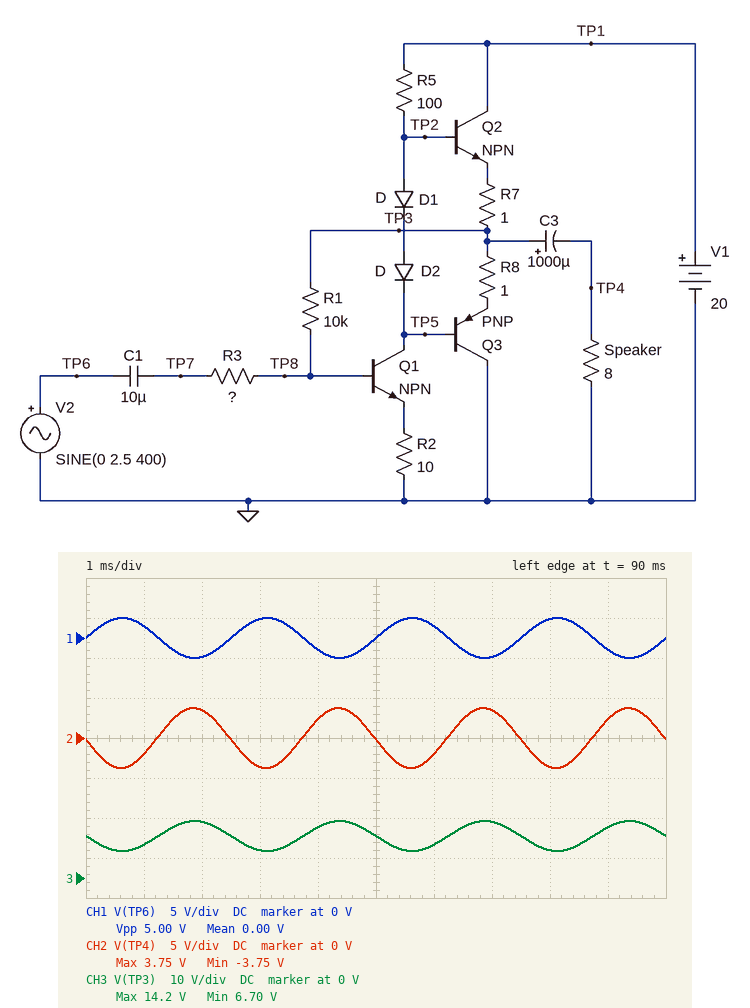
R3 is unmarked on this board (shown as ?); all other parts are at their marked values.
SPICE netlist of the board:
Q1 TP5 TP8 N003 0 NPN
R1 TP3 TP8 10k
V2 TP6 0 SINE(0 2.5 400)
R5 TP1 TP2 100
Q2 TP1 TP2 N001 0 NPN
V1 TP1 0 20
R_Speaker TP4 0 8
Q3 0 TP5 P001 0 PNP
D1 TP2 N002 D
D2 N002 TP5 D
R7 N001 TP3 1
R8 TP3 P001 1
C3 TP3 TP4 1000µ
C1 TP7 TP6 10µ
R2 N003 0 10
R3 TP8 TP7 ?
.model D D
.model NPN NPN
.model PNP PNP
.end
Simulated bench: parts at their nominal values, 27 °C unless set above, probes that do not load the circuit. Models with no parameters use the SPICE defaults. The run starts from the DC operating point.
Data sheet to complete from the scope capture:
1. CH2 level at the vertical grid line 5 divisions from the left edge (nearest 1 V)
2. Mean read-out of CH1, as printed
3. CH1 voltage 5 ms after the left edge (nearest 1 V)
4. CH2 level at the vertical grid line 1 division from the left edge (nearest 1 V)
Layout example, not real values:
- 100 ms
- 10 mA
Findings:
- 0 V
- 0.00 V
- 0 V
- -2 V
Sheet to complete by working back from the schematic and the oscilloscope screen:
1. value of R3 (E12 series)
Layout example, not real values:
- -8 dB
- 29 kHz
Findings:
- 2.2 kΩ
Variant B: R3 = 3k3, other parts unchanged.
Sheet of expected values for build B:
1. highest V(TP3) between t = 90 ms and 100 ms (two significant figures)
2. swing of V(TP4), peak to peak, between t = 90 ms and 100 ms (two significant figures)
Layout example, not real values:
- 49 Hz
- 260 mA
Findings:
- 13 V
- 5.3 V
